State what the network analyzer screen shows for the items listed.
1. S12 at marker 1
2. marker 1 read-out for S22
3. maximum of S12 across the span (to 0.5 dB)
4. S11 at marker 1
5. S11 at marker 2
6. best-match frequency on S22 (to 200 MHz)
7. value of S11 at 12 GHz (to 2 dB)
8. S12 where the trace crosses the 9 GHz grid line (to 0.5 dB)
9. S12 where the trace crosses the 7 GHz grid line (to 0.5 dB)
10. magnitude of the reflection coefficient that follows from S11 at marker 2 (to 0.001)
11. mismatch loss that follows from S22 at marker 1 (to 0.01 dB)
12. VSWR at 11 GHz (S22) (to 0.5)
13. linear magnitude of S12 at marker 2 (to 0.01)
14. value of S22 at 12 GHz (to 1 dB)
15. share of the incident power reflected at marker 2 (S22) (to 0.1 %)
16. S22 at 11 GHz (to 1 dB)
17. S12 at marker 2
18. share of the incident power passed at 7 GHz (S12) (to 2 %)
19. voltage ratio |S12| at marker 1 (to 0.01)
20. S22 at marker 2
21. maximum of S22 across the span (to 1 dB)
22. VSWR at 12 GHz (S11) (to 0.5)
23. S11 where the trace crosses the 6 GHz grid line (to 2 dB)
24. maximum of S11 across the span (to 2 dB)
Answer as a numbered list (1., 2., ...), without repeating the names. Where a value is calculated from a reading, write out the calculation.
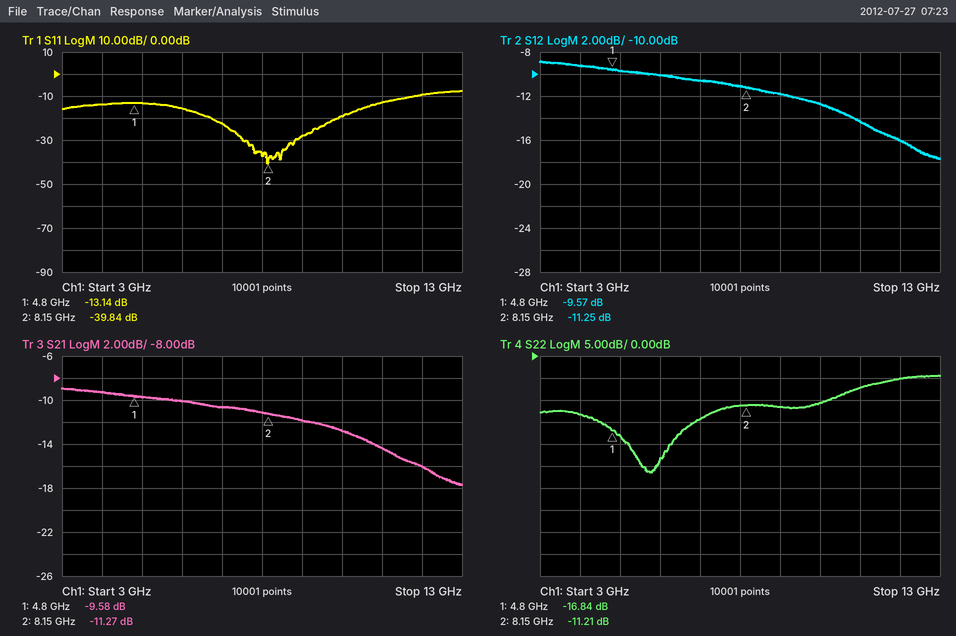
1. -9.57 dB
2. -16.84 dB
3. -9.0 dB
4. -13.14 dB
5. -39.84 dB
6. 5.8 GHz
7. -10 dB
8. -12.0 dB
9. -10.5 dB
10. 10^(-39.84/20) ≈ 0.010
11. −10 log10(1 − 10^(-16.84/10)) ≈ 0.09 dB
12. |Γ| = 10^(-7/20) = 0.4467; VSWR = (1 + 0.4467)/(1 − 0.4467) ≈ 2.61, so 2.5 to the nearest 0.5
13. 10^(-11.25/20) ≈ 0.27
14. -5 dB
15. 10^(-11.21/10) ≈ 7.6 %
16. -7 dB
17. -11.25 dB
18. 10^(-10.5/10) ≈ 8.91 %, so 8 % to the nearest 2 %
19. 10^(-9.57/20) ≈ 0.33
20. -11.21 dB
21. -4 dB
22. |Γ| = 10^(-10/20) = 0.3162; VSWR = (1 + 0.3162)/(1 − 0.3162) ≈ 1.92, so 2.0 to the nearest 0.5
23. -16 dB
24. -8 dB
